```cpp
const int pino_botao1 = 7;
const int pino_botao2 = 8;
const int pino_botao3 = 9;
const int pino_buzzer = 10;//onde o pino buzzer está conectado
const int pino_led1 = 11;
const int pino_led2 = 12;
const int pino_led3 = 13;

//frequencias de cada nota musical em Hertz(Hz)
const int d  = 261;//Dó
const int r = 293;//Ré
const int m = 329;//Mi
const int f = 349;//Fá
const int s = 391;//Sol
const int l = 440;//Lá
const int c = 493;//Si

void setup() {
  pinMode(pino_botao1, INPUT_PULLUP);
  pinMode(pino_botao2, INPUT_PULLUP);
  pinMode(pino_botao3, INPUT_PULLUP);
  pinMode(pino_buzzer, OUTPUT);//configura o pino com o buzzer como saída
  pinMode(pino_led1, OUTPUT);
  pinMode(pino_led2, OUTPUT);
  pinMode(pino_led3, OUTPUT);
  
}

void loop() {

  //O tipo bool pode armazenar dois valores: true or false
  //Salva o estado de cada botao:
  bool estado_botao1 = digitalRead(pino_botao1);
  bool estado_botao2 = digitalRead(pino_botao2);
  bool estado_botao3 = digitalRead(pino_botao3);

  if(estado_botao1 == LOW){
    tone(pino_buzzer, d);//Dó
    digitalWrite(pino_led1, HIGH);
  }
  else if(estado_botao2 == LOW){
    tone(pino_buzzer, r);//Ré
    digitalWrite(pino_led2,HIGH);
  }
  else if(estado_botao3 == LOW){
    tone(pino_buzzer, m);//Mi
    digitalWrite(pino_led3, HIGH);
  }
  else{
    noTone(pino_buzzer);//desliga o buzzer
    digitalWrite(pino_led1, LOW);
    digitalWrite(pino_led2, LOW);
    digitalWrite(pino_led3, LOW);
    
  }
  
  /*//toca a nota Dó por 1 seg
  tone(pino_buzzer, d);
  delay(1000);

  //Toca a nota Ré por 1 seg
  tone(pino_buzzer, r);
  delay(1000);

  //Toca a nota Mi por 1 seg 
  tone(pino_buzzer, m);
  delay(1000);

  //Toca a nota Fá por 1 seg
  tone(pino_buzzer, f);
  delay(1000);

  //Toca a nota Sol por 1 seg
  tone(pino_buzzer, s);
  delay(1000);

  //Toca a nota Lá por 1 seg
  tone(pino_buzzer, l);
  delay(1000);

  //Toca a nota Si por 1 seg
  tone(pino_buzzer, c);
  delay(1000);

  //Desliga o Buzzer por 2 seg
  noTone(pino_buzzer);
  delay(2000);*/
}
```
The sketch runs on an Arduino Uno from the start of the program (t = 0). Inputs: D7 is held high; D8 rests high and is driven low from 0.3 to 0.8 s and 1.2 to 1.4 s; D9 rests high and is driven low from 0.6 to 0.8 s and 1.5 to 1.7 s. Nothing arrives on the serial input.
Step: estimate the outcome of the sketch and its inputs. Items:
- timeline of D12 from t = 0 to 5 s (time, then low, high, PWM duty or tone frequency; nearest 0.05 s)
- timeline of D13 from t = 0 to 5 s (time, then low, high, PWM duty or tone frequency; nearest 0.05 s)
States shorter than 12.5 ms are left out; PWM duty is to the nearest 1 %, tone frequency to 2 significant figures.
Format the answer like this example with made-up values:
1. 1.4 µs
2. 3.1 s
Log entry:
1. 0 s low; 0.3 s high; 0.8 s low; 1.2 s high; 1.4 s low
2. 0 s low; 1.5 s high; 1.7 s low
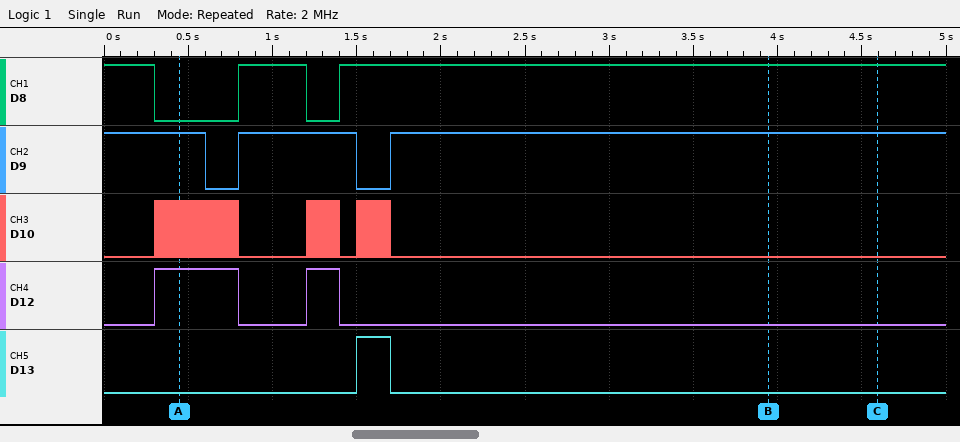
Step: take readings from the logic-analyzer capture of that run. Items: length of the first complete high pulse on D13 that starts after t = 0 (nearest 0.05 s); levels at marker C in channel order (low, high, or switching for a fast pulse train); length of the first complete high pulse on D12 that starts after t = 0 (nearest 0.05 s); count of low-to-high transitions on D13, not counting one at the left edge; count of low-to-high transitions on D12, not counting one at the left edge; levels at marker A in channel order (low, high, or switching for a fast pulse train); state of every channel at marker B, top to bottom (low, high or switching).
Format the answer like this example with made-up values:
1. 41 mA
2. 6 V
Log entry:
1. 0.20 s
2. D8 high, D9 high, D10 low, D12 low, D13 low
3. 0.50 s
4. 1
5. 2
6. D8 low, D9 high, D10 switching, D12 high, D13 low
7. D8 high, D9 high, D10 low, D12 low, D13 low
